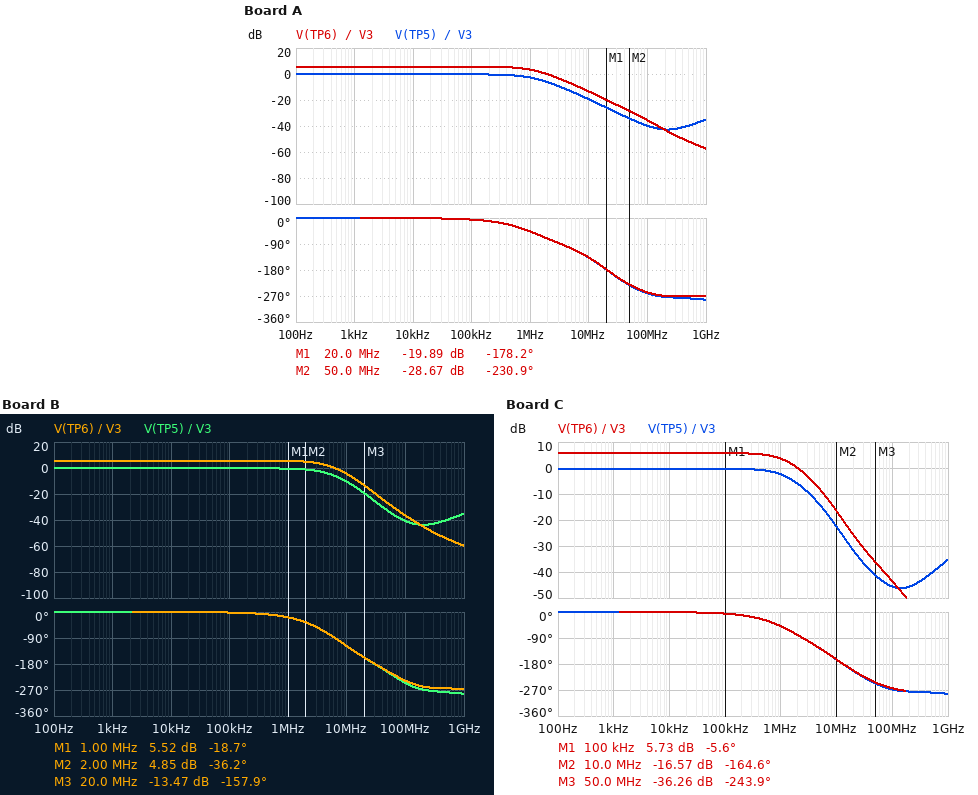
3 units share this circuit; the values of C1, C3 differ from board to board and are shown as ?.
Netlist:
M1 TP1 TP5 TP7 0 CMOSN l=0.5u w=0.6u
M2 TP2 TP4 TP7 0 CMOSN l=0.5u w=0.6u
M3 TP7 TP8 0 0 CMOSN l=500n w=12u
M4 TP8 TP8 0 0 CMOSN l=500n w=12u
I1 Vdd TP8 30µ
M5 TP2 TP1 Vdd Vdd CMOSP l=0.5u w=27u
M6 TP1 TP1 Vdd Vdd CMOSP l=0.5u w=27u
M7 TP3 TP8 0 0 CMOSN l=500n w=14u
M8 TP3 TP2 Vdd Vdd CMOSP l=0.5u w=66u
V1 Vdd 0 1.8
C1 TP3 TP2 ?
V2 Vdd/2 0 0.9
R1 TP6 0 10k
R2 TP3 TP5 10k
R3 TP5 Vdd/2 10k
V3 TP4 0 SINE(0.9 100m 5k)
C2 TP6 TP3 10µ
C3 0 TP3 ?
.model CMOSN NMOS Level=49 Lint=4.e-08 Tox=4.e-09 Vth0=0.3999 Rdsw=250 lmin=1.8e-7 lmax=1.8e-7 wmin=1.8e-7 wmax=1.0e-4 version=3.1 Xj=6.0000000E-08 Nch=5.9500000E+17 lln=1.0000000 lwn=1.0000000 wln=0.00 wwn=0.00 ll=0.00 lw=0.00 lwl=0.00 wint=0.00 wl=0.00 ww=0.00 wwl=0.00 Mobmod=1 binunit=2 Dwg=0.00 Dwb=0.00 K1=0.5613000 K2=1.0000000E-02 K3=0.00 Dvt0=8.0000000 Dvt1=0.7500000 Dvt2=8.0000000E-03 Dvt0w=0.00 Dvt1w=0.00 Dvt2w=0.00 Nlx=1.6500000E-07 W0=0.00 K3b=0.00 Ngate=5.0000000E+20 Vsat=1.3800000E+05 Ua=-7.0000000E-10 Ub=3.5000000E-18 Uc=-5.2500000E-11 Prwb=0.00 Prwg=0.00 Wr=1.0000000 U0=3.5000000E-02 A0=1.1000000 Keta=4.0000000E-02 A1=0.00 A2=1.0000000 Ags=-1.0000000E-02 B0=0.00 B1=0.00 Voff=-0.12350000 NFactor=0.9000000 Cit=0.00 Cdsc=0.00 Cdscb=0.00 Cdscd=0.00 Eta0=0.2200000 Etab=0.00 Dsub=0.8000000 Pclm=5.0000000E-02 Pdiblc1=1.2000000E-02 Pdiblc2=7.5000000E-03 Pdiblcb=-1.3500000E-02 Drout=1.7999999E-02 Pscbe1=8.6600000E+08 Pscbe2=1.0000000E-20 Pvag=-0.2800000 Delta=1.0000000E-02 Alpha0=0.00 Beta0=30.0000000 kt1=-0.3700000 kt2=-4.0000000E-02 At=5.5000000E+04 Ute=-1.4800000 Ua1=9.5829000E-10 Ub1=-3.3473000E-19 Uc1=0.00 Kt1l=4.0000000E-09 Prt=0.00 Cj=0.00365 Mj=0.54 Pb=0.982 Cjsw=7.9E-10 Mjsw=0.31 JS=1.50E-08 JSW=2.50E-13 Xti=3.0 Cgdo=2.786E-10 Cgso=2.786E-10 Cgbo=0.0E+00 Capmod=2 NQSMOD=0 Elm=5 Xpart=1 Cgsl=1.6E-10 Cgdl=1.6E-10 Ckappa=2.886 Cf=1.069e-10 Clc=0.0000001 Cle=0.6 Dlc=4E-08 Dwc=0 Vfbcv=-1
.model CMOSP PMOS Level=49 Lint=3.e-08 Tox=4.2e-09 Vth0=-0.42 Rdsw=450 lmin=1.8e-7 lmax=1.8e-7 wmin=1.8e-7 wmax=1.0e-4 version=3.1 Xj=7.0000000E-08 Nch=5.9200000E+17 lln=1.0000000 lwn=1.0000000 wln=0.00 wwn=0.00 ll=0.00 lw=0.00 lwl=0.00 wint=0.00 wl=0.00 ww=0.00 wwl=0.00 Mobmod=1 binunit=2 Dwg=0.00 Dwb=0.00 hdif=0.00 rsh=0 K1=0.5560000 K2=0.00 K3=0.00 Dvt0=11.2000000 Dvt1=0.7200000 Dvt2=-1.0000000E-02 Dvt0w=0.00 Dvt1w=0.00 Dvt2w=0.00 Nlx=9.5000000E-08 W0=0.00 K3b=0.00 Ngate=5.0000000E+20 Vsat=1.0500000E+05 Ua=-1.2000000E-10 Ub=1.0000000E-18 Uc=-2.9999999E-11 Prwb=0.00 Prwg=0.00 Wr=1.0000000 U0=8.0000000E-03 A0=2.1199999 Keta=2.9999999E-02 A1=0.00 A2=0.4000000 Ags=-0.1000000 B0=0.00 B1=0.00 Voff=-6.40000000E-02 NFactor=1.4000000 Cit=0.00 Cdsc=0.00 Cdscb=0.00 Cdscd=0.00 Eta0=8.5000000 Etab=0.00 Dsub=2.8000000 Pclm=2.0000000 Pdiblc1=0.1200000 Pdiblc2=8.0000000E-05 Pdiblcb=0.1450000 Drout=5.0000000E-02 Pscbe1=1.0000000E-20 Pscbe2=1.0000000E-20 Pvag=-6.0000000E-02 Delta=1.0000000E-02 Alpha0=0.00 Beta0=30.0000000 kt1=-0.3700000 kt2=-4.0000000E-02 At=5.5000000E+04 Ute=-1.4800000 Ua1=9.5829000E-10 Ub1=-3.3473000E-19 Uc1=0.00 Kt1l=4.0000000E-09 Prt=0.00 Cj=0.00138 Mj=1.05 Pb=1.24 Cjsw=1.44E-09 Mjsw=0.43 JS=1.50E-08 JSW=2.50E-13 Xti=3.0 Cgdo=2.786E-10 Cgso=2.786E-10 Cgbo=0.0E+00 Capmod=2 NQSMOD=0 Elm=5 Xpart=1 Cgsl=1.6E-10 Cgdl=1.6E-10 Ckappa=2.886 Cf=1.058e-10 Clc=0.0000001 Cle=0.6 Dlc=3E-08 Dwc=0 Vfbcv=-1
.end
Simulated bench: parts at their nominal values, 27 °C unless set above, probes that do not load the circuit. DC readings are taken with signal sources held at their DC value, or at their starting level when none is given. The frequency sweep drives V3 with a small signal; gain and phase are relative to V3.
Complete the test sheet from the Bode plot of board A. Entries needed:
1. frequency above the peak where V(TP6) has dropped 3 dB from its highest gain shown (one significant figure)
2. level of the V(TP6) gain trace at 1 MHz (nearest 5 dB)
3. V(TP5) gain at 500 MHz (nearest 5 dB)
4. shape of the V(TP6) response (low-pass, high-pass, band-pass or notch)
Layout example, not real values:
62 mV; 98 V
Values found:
1 MHz; 5 dB; -40 dB; low-pass
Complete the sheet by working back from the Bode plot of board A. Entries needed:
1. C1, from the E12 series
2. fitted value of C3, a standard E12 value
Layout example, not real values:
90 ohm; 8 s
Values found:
4.7 pF; 5.6 pF
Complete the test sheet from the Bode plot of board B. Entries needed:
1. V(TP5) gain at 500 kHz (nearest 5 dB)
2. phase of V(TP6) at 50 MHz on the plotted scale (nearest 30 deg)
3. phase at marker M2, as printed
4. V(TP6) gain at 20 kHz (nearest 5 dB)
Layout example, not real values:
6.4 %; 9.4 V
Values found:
0 dB; -210 deg; -36.2 deg; 5 dB
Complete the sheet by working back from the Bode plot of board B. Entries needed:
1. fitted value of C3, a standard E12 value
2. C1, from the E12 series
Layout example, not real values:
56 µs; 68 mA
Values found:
6.8 pF; 1.5 pF
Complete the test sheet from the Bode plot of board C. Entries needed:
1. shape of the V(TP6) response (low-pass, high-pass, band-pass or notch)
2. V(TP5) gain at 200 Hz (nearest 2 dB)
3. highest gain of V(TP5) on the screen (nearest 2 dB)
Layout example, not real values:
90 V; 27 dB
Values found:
low-pass; 0 dB; 0 dB
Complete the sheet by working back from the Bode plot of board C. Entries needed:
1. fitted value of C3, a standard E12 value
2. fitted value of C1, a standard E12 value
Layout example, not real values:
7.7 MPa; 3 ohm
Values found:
15 pF; 4.7 pF
